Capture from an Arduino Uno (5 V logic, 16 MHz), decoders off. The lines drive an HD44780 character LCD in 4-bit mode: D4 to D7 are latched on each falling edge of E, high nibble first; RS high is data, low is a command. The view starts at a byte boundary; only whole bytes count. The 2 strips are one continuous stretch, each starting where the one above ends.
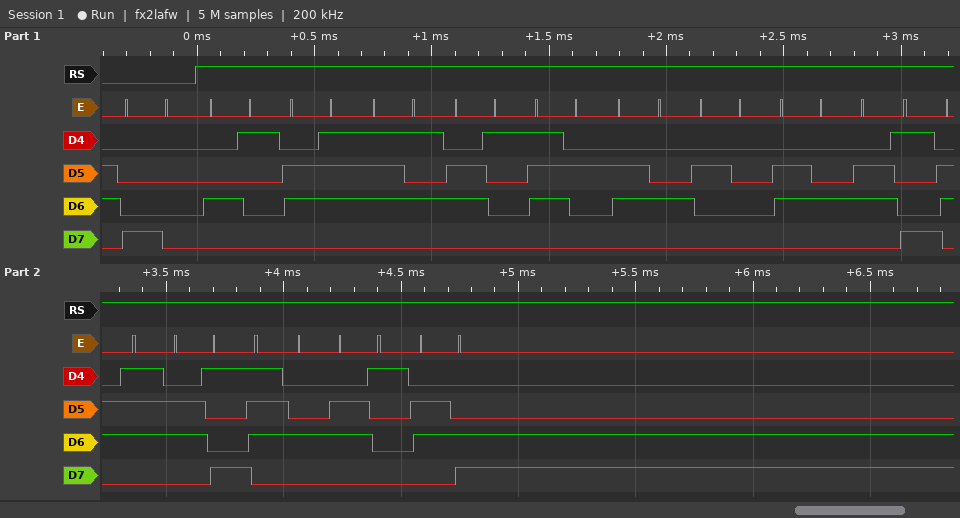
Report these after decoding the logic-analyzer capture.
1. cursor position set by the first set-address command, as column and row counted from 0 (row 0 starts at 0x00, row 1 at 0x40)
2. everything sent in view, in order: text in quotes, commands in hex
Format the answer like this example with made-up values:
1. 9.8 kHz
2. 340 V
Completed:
1. column 0, row 0
2. 0x80 "Aguard digital"
